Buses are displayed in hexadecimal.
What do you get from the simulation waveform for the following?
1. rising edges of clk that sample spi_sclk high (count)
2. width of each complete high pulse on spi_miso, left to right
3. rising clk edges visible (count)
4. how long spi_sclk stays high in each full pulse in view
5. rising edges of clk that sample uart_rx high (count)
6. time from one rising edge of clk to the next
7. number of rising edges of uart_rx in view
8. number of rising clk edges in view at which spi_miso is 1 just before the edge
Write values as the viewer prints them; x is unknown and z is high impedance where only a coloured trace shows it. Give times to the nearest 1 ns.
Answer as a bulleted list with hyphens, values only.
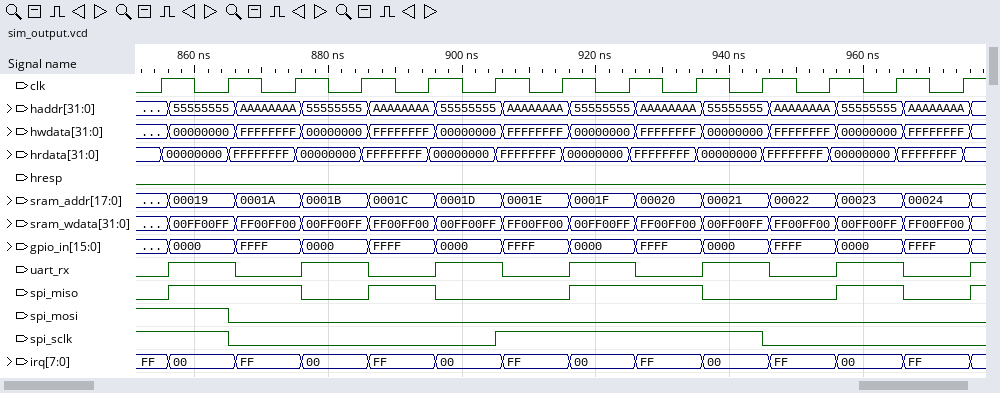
- 6
- 20 ns, 10 ns, 20 ns, 10 ns
- 13
- 40 ns
- 6
- 10 ns
- 7
- 6
